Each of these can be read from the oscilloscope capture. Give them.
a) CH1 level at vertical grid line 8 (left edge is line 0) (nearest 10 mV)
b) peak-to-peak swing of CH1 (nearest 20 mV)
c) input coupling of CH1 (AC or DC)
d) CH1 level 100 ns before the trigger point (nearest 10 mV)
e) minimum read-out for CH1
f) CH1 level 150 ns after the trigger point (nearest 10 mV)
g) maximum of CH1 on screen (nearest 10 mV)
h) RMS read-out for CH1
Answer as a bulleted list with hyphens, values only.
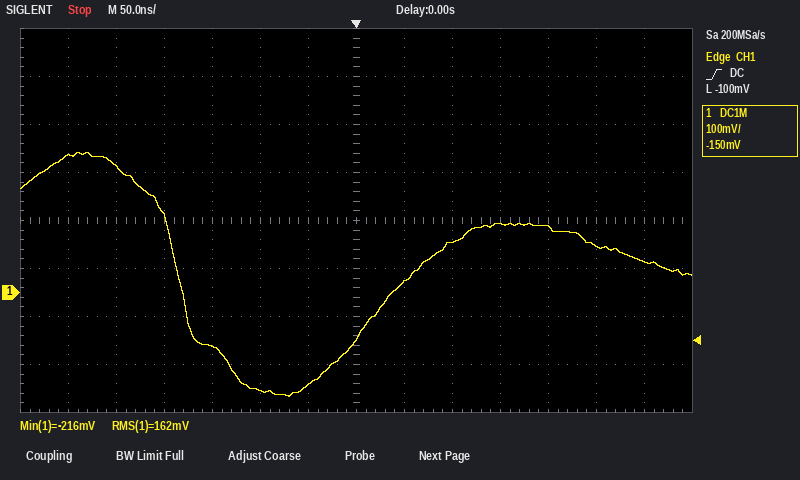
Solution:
- 20 mV
- 500 mV
- DC
- -200 mV
- -216 mV
- 140 mV
- 290 mV
- 162 mV
